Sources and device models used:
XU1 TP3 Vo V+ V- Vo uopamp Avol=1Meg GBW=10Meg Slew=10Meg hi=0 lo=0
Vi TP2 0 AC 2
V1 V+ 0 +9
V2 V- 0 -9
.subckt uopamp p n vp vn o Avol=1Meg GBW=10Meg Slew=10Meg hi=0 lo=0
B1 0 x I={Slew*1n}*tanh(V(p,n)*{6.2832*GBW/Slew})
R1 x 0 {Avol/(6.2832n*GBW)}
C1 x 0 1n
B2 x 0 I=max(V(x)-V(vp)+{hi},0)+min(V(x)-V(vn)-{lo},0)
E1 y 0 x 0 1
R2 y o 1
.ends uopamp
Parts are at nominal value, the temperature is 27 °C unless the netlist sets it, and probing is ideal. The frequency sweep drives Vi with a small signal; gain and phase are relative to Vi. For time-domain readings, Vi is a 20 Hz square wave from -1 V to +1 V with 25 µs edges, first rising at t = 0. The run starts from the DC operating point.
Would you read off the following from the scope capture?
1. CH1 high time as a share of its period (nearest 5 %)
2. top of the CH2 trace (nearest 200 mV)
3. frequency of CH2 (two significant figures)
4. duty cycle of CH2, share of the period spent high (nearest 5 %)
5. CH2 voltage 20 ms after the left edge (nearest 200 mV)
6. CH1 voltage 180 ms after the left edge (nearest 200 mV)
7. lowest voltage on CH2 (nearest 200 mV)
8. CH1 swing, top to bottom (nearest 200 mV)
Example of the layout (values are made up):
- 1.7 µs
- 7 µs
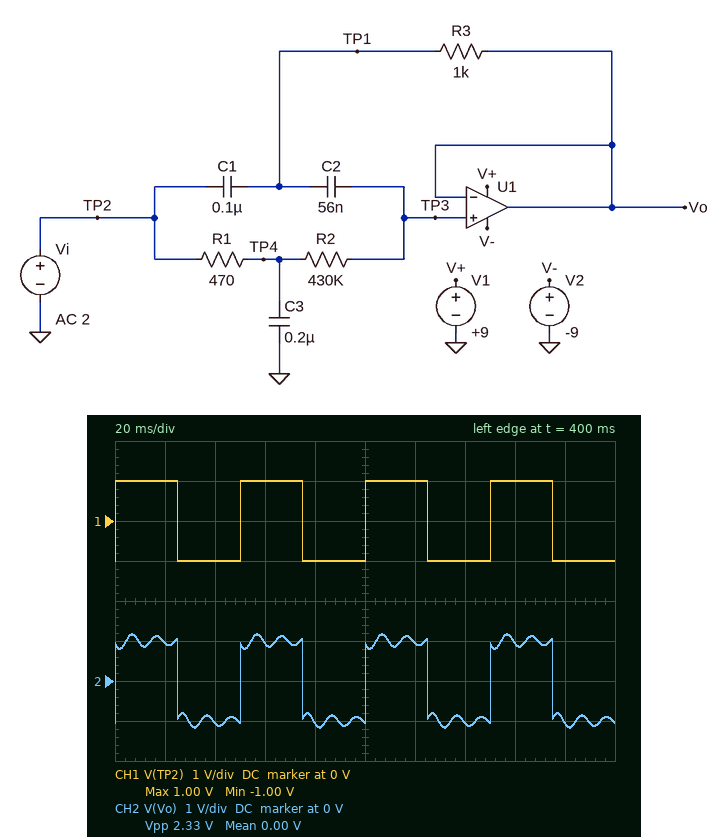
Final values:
- 50 %
- 1.2 V
- 20 Hz
- 50 %
- 1.0 V
- -1.0 V
- -1.2 V
- 2.0 V
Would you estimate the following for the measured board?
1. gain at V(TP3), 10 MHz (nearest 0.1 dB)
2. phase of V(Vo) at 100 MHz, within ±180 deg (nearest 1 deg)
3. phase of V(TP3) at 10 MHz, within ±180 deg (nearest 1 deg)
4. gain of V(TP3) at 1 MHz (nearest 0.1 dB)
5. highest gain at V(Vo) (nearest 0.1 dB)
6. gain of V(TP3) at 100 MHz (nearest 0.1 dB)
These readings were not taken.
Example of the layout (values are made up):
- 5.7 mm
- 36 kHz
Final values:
- 0 dB
- -84 deg
- 0 deg
- 0 dB
- 0 dB
- 0 dB
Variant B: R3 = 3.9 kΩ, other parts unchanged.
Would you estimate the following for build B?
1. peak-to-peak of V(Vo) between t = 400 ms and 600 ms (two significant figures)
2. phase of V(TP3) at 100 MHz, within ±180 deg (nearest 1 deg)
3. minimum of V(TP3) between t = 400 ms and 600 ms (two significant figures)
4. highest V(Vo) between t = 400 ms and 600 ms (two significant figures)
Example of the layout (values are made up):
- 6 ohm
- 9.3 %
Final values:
- 2.1 V
- 0 deg
- -1.0 V
- 1.0 V
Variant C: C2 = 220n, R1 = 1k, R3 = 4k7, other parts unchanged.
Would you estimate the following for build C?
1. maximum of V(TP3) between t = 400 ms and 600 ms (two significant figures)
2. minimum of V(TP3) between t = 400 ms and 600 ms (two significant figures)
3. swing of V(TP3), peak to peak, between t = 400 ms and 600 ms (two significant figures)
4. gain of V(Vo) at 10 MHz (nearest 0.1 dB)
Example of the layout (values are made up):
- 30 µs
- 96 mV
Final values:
- 1.1 V
- -1.1 V
- 2.1 V
- -3.0 dB
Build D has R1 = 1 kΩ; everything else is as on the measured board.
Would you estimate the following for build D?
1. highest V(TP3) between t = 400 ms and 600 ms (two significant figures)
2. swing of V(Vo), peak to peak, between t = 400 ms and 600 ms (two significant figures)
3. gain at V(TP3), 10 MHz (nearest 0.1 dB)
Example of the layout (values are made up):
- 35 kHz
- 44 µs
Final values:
- 1.3 V
- 2.7 V
- 0 dB
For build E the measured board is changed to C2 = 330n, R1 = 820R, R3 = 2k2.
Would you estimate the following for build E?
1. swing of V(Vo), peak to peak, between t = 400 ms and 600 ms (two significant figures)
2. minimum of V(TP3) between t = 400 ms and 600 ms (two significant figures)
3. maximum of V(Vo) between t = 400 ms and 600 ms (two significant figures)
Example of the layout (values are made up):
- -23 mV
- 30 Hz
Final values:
- 2.1 V
- -1.0 V
- 1.0 V
